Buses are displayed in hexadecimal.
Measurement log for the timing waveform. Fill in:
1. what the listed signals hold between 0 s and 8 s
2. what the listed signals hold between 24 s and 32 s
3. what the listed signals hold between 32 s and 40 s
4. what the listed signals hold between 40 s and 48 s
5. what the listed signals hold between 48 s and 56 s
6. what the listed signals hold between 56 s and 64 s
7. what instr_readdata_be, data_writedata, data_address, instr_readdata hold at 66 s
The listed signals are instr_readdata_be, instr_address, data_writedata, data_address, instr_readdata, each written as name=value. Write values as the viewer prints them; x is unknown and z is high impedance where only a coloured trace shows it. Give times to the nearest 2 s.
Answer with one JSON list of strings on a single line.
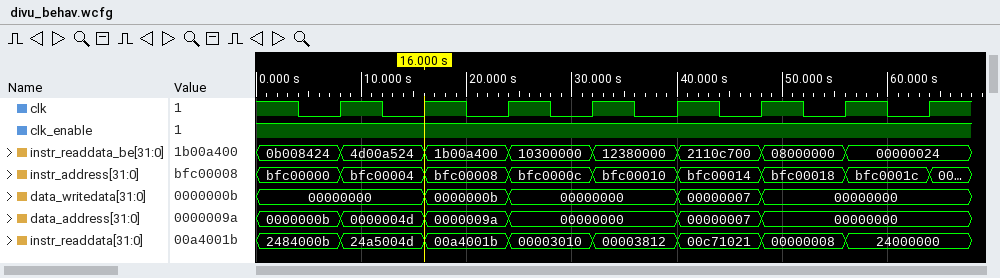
["instr_readdata_be=0b008424, instr_address=bfc00000, data_writedata=00000000, data_address=0000000b, instr_readdata=2484000b", "instr_readdata_be=10300000, instr_address=bfc0000c, data_writedata=00000000, data_address=00000000, instr_readdata=00003010", "instr_readdata_be=12380000, instr_address=bfc00010, data_writedata=00000000, data_address=00000000, instr_readdata=00003812", "instr_readdata_be=2110c700, instr_address=bfc00014, data_writedata=00000007, data_address=00000007, instr_readdata=00c71021", "instr_readdata_be=08000000, instr_address=bfc00018, data_writedata=00000000, data_address=00000000, instr_readdata=00000008", "instr_readdata_be=00000024, instr_address=bfc0001c, data_writedata=00000000, data_address=00000000, instr_readdata=24000000", "instr_readdata_be=00000024, data_writedata=00000000, data_address=00000000, instr_readdata=24000000"]
